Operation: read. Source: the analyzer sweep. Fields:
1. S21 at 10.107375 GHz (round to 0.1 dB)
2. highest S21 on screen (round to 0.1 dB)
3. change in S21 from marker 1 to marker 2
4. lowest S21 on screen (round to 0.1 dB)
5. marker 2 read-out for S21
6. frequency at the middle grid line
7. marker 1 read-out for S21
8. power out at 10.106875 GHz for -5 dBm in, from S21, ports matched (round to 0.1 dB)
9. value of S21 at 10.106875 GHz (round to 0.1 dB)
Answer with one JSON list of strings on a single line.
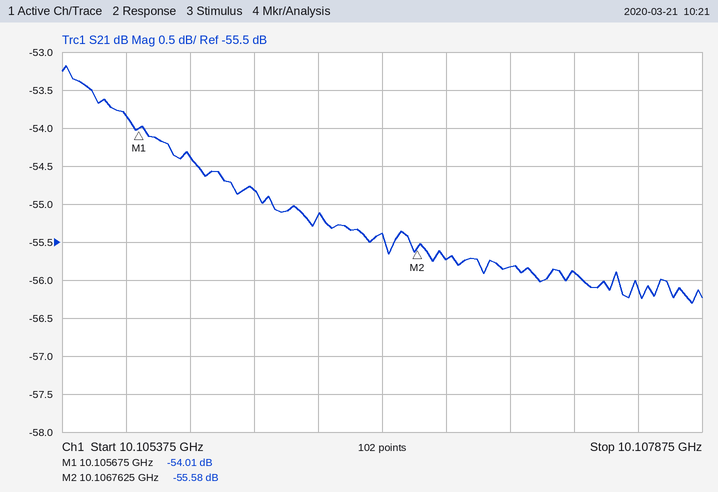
["-55.9 dB", "-53.2 dB", "-1.57 dB", "-56.3 dB", "-55.58 dB", "10.106625 GHz", "-54.01 dB", "-60.7 dBm", "-55.7 dB"]
